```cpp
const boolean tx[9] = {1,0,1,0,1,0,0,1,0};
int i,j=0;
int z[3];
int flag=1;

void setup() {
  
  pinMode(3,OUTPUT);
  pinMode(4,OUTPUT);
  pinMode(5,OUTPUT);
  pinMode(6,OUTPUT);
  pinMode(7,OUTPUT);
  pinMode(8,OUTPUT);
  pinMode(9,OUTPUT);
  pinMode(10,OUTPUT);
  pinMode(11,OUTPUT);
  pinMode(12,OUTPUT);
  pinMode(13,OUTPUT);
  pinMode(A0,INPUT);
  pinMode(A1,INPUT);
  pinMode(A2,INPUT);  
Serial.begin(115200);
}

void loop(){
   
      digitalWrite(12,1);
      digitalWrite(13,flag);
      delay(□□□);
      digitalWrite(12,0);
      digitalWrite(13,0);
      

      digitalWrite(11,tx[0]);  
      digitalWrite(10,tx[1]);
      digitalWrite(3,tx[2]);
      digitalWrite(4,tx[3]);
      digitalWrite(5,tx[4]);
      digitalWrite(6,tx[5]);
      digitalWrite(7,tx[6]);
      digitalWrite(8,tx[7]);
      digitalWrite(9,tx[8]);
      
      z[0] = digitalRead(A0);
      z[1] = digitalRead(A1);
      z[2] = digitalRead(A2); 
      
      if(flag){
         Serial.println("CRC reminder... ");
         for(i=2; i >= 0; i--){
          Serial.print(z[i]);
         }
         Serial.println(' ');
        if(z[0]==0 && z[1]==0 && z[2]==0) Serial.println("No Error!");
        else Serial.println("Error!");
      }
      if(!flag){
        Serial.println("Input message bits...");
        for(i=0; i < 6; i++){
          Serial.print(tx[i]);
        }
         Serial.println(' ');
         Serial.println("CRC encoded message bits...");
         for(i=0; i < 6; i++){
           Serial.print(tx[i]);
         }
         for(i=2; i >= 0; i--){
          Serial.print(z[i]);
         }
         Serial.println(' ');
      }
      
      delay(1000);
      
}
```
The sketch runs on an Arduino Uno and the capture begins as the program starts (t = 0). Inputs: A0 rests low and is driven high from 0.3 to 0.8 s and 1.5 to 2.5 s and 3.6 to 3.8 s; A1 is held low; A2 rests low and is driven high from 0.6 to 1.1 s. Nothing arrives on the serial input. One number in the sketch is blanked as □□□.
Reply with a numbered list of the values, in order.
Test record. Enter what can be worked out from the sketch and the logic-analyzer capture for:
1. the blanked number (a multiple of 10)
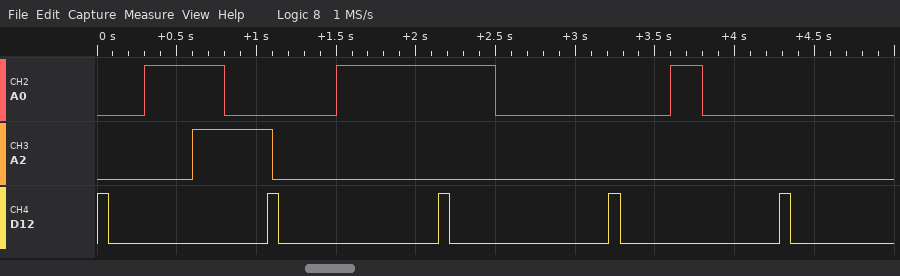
1. 70
